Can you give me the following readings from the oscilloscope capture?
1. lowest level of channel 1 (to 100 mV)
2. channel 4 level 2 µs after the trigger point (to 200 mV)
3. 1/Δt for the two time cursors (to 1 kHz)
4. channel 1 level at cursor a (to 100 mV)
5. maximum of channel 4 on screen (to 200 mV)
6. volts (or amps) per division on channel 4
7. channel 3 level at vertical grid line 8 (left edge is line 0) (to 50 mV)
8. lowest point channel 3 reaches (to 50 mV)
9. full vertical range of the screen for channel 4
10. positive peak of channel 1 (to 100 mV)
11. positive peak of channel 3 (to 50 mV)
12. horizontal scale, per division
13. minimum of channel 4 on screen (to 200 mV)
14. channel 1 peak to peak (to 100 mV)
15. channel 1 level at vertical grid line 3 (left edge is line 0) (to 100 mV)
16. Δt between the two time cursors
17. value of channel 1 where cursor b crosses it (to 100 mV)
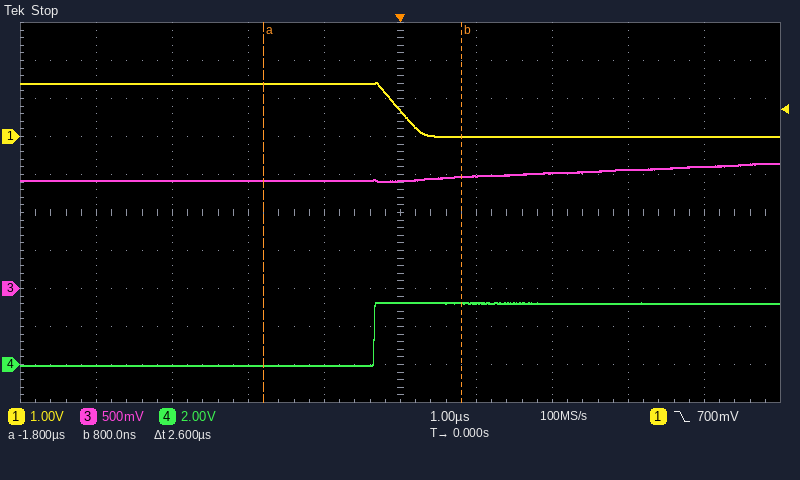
0.0 V
3.2 V
385 kHz
1.4 V
3.2 V
2 V
1.55 V
1.40 V
20 V
1.4 V
1.65 V
1 µs
0.0 V
1.4 V
1.4 V
2.6 µs
0.0 V
